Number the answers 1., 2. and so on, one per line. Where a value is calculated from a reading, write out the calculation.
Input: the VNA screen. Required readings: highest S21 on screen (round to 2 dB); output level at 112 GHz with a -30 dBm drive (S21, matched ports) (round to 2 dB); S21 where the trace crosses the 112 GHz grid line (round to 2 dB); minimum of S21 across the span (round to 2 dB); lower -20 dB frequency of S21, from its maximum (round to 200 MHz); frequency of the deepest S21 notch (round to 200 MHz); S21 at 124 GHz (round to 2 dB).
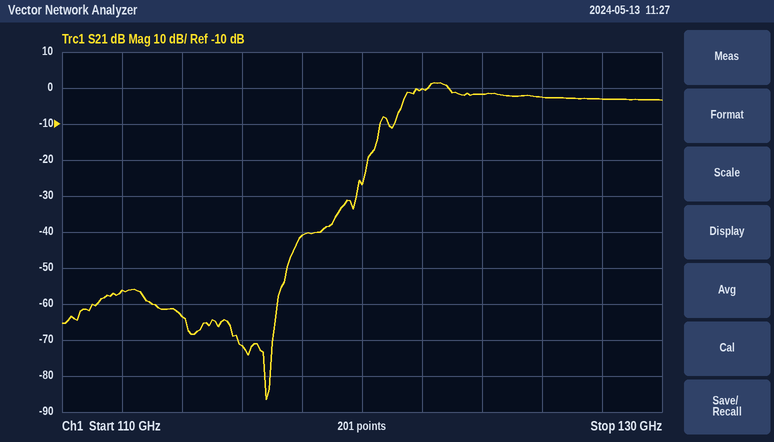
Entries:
1. 2 dB
2. -30 dBm + (-56 dB) = -86 dBm
3. -56 dB
4. -86 dB
5. 120.2 GHz
6. 116.8 GHz
7. -2 dB
